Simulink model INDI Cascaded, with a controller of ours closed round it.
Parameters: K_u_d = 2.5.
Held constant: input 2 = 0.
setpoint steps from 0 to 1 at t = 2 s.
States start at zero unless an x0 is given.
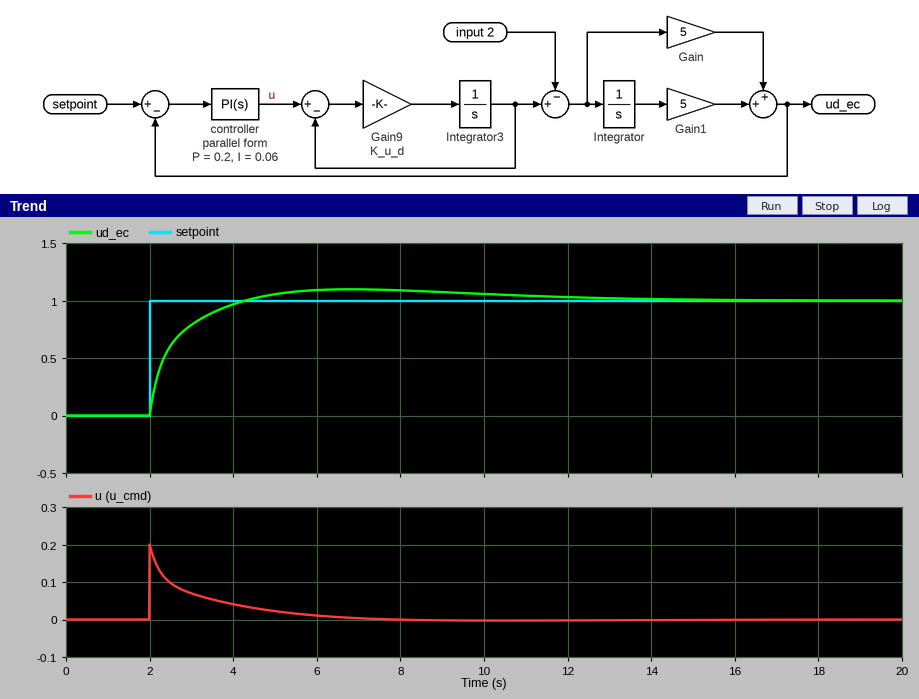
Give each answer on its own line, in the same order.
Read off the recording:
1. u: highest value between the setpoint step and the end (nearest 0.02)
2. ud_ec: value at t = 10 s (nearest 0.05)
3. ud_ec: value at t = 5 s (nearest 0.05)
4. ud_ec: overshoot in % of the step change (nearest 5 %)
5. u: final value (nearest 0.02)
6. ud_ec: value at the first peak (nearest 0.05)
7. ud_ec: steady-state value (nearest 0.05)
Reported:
0.20
1.05
1.05
10 %
0.00
1.10
1.00
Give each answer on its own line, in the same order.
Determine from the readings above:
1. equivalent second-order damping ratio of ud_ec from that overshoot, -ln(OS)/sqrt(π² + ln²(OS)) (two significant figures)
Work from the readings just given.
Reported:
0.59
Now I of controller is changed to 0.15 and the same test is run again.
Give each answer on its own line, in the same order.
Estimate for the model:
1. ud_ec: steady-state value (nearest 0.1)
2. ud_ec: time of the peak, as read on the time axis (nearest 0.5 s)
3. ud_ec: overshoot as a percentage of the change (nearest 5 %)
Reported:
1.0
5.0 s
15 %
